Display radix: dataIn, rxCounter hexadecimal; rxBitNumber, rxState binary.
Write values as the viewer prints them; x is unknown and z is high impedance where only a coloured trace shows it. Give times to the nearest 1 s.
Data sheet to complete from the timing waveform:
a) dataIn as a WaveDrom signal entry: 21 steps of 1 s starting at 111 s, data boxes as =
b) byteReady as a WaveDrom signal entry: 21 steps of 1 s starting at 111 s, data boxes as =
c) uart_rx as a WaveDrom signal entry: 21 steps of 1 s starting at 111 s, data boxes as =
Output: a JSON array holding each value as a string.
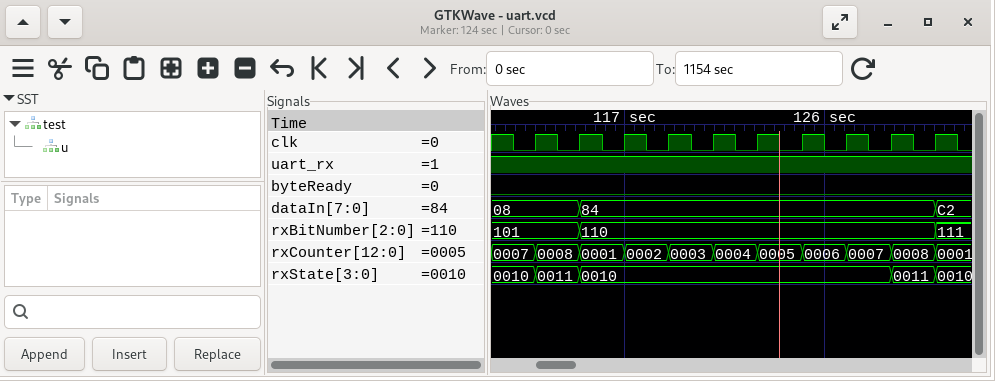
["{name: 'dataIn', wave: '=...=...............=', data: '08 84 C2'}", "{name: 'byteReady', wave: '0....................'}", "{name: 'uart_rx', wave: '1....................'}"]
